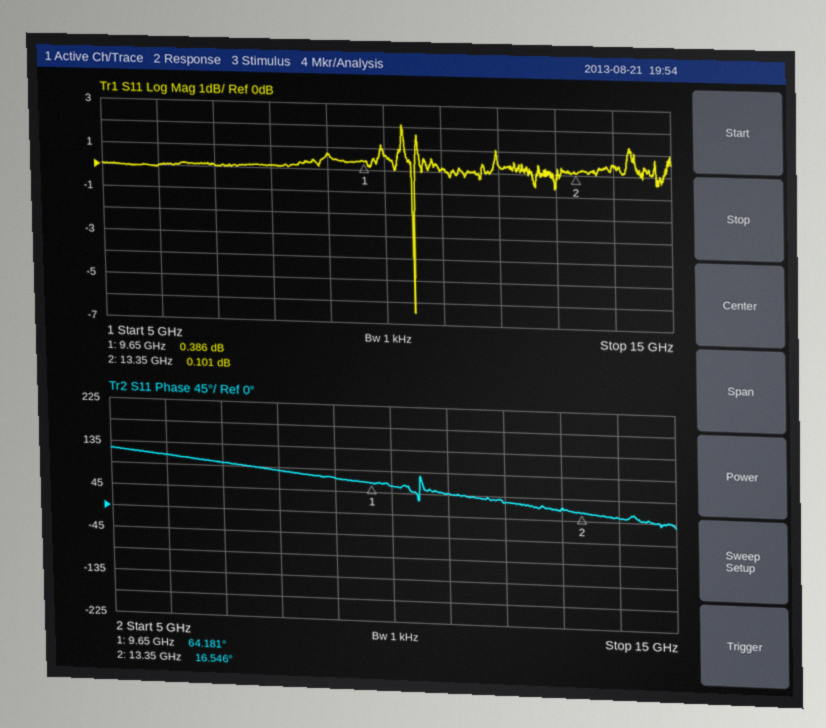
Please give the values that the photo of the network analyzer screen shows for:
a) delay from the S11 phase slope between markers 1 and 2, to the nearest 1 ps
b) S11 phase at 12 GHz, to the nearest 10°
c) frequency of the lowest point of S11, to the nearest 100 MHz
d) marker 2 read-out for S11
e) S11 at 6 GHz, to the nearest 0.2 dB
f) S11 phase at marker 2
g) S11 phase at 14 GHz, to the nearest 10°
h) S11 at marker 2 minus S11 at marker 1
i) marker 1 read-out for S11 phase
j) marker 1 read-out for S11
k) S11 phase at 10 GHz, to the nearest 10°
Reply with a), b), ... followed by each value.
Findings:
a) 36 ps
b) 30°
c) 10.5 GHz
d) 0.101 dB
e) 0.0 dB
f) 16.546°
g) 10°
h) -0.285 dB
i) 64.181°
j) 0.386 dB
k) 60°
